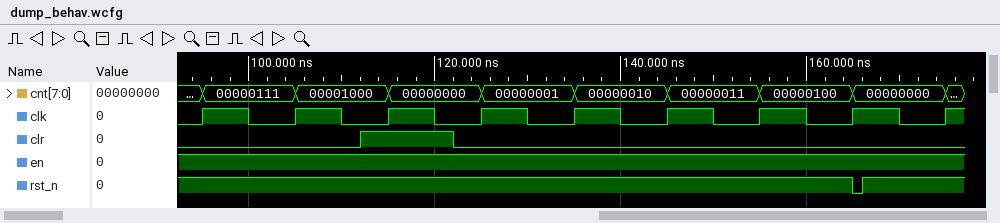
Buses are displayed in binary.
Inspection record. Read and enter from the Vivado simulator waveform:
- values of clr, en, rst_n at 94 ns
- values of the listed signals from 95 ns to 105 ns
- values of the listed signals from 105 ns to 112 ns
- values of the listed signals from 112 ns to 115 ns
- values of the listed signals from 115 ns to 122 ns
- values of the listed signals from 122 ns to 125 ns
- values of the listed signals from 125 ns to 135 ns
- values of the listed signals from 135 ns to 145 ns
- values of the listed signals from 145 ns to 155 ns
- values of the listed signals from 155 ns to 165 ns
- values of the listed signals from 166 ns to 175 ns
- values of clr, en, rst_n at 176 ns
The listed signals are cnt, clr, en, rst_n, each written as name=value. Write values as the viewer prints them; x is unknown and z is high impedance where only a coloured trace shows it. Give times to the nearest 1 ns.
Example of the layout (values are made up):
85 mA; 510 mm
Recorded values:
clr=0, en=1, rst_n=1; cnt=00000111, clr=0, en=1, rst_n=1; cnt=00001000, clr=0, en=1, rst_n=1; cnt=00001000, clr=1, en=1, rst_n=1; cnt=00000000, clr=1, en=1, rst_n=1; cnt=00000000, clr=0, en=1, rst_n=1; cnt=00000001, clr=0, en=1, rst_n=1; cnt=00000010, clr=0, en=1, rst_n=1; cnt=00000011, clr=0, en=1, rst_n=1; cnt=00000100, clr=0, en=1, rst_n=1; cnt=00000000, clr=0, en=1, rst_n=1; clr=0, en=1, rst_n=1
